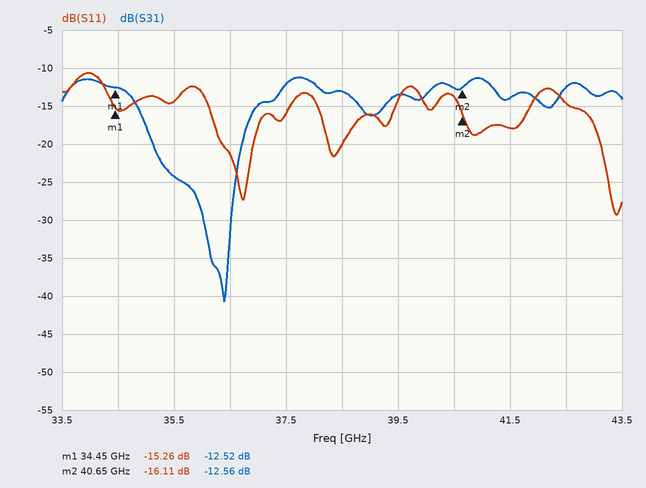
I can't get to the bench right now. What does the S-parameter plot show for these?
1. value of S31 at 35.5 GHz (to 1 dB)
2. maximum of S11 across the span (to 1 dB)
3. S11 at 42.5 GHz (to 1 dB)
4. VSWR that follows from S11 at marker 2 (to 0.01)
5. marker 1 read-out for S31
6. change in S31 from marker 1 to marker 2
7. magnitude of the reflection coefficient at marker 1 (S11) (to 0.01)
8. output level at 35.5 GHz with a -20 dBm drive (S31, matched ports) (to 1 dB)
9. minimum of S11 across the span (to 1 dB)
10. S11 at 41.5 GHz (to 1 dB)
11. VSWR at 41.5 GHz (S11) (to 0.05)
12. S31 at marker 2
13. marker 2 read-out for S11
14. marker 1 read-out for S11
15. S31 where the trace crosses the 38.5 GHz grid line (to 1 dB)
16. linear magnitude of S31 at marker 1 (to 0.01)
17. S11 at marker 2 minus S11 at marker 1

-24 dB
-11 dB
-15 dB
1.37
-12.52 dB
-0.04 dB
0.17
-44 dBm
-29 dB
-18 dB
1.30
-12.56 dB
-16.11 dB
-15.26 dB
-13 dB
0.24
-0.85 dB
